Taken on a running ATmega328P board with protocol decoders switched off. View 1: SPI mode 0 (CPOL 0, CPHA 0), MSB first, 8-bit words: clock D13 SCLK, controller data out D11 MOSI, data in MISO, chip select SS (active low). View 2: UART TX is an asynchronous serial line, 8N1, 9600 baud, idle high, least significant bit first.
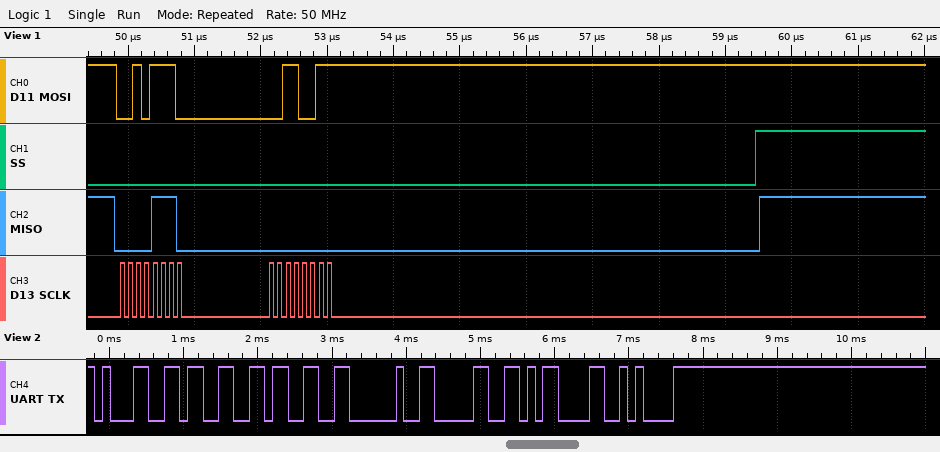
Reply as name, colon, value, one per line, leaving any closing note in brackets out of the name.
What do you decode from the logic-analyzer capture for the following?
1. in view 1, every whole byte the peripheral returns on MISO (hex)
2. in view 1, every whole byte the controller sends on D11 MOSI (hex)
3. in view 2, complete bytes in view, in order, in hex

in view 1, every whole byte the peripheral returns on MISO: 0E 00
in view 1, every whole byte the controller sends on D11 MOSI: 2E 33
in view 2, complete bytes in view, in order, in hex: 31 33 33 20 30 0D 0A
